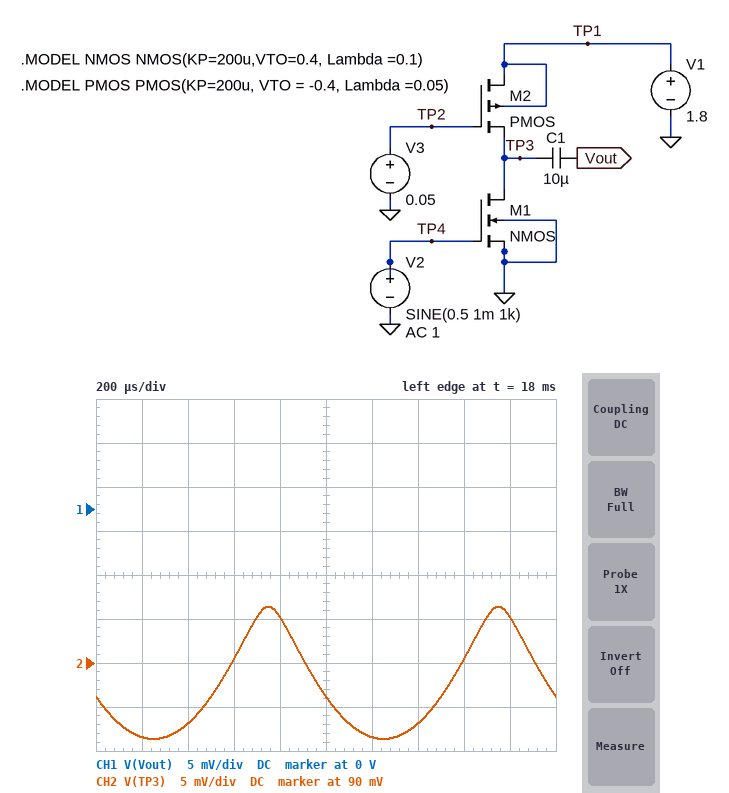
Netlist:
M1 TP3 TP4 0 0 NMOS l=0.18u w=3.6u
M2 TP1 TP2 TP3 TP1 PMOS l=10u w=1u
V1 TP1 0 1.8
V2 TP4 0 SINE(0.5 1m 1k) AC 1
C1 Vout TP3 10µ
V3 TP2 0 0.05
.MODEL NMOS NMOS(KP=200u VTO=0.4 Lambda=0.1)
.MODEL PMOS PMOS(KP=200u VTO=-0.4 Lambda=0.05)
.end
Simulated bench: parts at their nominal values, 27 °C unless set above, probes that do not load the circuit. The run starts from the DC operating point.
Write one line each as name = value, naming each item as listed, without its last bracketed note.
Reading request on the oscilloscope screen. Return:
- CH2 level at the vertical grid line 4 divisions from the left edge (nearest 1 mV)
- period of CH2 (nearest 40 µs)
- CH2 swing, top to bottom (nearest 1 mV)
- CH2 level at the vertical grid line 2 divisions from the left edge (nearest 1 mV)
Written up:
CH2 level at the vertical grid line 4 divisions from the left edge = 95 mV
period of CH2 = 1.00 ms
CH2 swing, top to bottom = 15 mV
CH2 level at the vertical grid line 2 divisions from the left edge = 83 mV
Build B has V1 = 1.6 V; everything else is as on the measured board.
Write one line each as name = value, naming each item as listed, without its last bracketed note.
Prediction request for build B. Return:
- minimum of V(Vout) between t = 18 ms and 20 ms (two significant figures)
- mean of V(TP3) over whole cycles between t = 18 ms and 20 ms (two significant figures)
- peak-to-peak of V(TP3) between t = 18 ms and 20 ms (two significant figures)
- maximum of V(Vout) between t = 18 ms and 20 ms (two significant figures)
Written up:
minimum of V(Vout) between t = 18 ms and 20 ms = 45 mV
mean of V(TP3) over whole cycles between t = 18 ms and 20 ms = 46 mV
peak-to-peak of V(TP3) between t = 18 ms and 20 ms = 1.7 mV
maximum of V(Vout) between t = 18 ms and 20 ms = 47 mV
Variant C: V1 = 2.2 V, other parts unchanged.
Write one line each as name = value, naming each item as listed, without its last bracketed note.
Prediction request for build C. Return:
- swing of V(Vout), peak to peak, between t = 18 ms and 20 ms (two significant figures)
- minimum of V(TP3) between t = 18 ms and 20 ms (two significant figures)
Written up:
swing of V(Vout), peak to peak, between t = 18 ms and 20 ms = 40 mV
minimum of V(TP3) between t = 18 ms and 20 ms = 1.4 V
